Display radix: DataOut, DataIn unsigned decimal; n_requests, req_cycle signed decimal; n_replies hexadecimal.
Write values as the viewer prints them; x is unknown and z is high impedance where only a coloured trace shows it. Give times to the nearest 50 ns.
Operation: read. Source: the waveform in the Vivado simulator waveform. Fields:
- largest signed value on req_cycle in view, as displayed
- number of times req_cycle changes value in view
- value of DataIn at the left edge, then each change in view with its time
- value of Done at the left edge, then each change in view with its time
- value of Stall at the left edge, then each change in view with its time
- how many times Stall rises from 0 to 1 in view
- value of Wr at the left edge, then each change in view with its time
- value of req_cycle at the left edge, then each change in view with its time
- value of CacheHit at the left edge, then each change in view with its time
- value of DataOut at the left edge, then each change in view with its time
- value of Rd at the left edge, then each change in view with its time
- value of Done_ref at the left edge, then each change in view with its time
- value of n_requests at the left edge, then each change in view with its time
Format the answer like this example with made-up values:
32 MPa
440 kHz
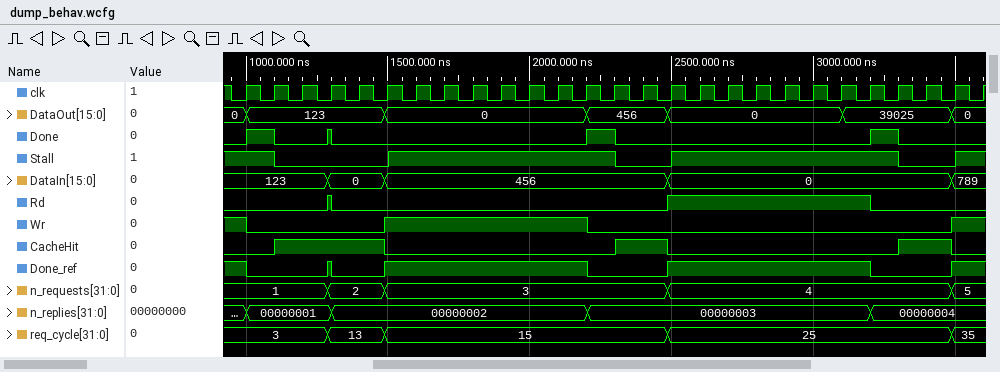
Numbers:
35
4
123, 0 at 1300 ns, 456 at 1500 ns, 0 at 2500 ns, 789 at 3500 ns
0, 1 at 1000 ns, 0 at 1100 ns, 1 at 1300 ns, 0 at 1300 ns, 1 at 2200 ns, 0 at 2300 ns, 1 at 3200 ns, 0 at 3300 ns
1, 0 at 1100 ns, 1 at 1500 ns, 0 at 2300 ns, 1 at 2500 ns, 0 at 3300 ns, 1 at 3500 ns
3
1, 0 at 1000 ns, 1 at 1500 ns, 0 at 2200 ns, 1 at 3500 ns
3, 13 at 1300 ns, 15 at 1500 ns, 25 at 2500 ns, 35 at 3500 ns
0, 1 at 1100 ns, 0 at 1500 ns, 1 at 2300 ns, 0 at 2500 ns, 1 at 3300 ns, 0 at 3500 ns
0, 123 at 1000 ns, 0 at 1500 ns, 456 at 2200 ns, 0 at 2500 ns, 39025 at 3100 ns, 0 at 3500 ns
0, 1 at 1300 ns, 0 at 1300 ns, 1 at 2500 ns, 0 at 3200 ns
1, 0 at 1000 ns, 1 at 1300 ns, 0 at 1300 ns, 1 at 1500 ns, 0 at 2200 ns, 1 at 2500 ns, 0 at 3200 ns, 1 at 3500 ns
1, 2 at 1300 ns, 3 at 1500 ns, 4 at 2500 ns, 5 at 3500 ns
